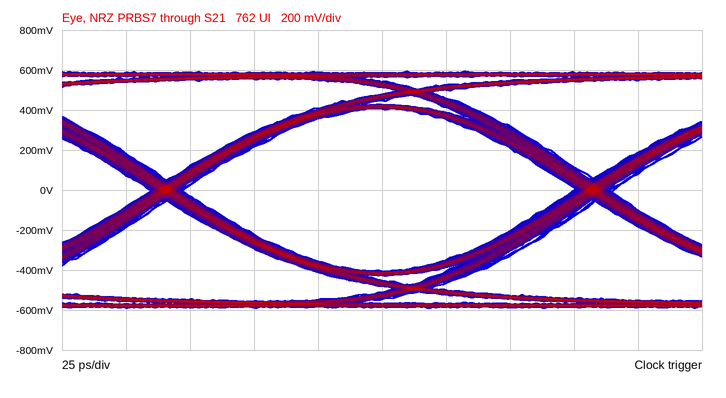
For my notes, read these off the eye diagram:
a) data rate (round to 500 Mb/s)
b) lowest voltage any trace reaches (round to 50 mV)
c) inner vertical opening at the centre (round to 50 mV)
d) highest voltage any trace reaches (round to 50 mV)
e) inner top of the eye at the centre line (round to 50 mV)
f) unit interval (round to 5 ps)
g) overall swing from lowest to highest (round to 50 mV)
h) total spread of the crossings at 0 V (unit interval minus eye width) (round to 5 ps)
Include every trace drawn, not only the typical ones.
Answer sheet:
6.0 Gb/s
-600 mV
800 mV
600 mV
400 mV
165 ps
1.20 V
15 ps
